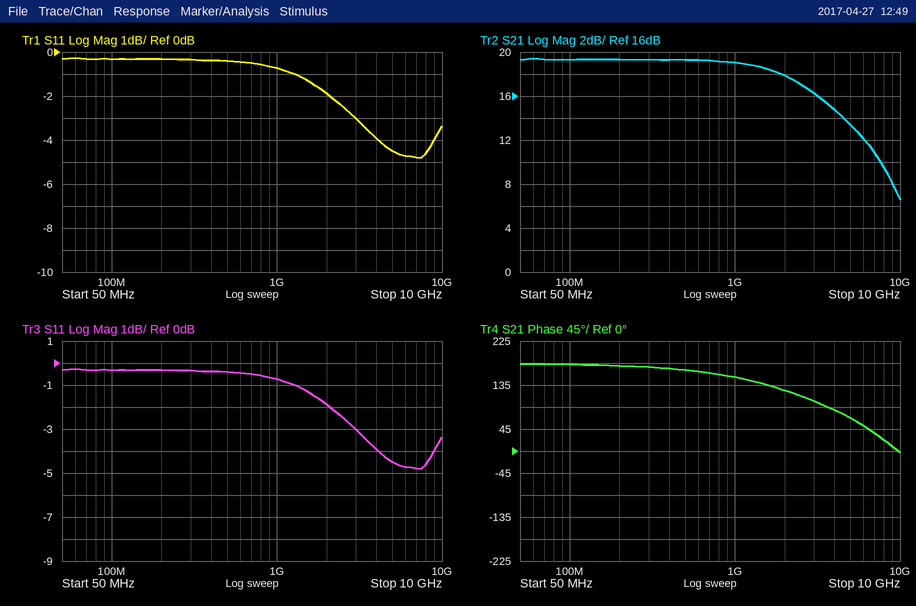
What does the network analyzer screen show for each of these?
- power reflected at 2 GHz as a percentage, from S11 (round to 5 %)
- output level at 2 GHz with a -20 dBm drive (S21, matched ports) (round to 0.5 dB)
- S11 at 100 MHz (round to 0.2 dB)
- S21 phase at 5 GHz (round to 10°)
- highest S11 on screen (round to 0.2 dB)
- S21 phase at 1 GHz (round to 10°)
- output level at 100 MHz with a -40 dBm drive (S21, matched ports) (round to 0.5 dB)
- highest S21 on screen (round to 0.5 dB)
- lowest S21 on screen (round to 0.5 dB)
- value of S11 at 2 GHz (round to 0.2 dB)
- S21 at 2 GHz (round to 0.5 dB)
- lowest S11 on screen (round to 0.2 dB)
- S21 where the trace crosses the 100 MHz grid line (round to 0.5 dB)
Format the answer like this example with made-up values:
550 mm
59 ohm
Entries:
65 %
-2.0 dBm
-0.4 dB
70°
-0.2 dB
150°
-20.5 dBm
19.5 dB
6.5 dB
-1.8 dB
18.0 dB
-4.8 dB
19.5 dB
